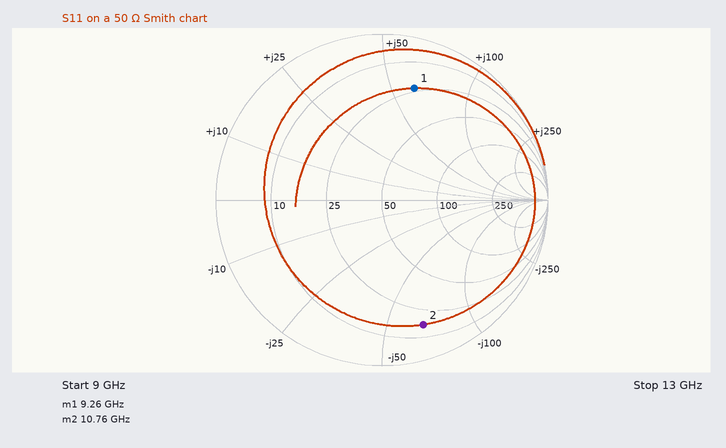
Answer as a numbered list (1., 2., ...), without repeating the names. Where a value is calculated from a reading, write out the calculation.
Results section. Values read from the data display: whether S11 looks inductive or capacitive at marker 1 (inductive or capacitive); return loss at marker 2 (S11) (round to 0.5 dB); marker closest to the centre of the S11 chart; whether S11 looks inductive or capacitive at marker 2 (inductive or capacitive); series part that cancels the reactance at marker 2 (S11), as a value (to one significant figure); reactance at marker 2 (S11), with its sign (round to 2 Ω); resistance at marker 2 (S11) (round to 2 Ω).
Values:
1. inductive
2. 2.0 dB
3. marker 1
4. capacitive
5. L = 66 Ω/(2π × 10.76 GHz) ≈ 1.0 nH
6. -66 Ω
7. 16 Ω
